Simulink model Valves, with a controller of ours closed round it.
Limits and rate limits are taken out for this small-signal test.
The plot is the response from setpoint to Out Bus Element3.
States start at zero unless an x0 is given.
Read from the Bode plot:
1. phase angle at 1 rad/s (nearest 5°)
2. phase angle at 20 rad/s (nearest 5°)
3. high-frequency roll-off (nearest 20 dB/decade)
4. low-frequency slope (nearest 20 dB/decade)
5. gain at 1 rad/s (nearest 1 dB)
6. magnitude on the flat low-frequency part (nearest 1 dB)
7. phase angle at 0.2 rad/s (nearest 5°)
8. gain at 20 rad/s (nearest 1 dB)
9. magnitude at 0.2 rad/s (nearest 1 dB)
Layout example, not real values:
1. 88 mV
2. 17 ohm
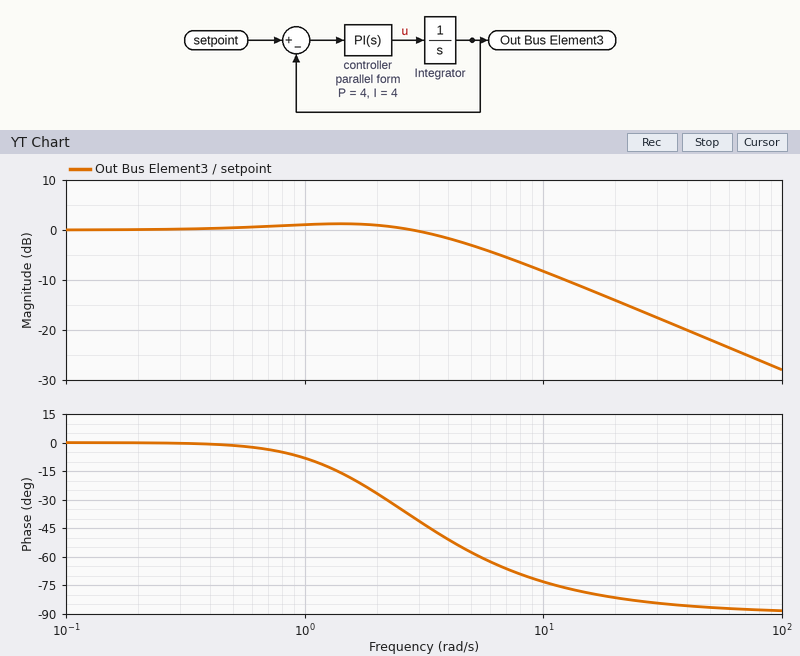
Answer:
1. -10°
2. -80°
3. -20 dB/decade
4. 0 dB/decade
5. 1 dB
6. 0 dB
7. 0°
8. -14 dB
9. 0 dB
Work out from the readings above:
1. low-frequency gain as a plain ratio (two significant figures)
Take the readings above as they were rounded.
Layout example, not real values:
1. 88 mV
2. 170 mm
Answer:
1. 1.0
